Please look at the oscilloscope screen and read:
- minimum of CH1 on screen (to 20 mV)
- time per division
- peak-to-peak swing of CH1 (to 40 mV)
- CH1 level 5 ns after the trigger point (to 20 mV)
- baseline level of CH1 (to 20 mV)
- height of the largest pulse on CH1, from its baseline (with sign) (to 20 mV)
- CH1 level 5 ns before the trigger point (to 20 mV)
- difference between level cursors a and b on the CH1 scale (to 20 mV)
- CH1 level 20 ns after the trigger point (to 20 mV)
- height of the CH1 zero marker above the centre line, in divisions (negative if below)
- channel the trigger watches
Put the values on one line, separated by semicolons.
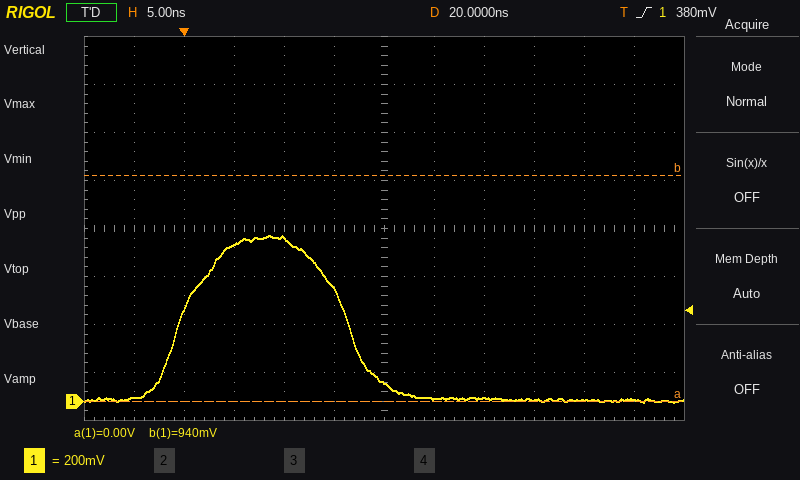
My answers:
0 mV; 5 ns; 680 mV; 660 mV; 0 mV; +680 mV; 20 mV; 940 mV; 80 mV; -3.6 div; CH1
